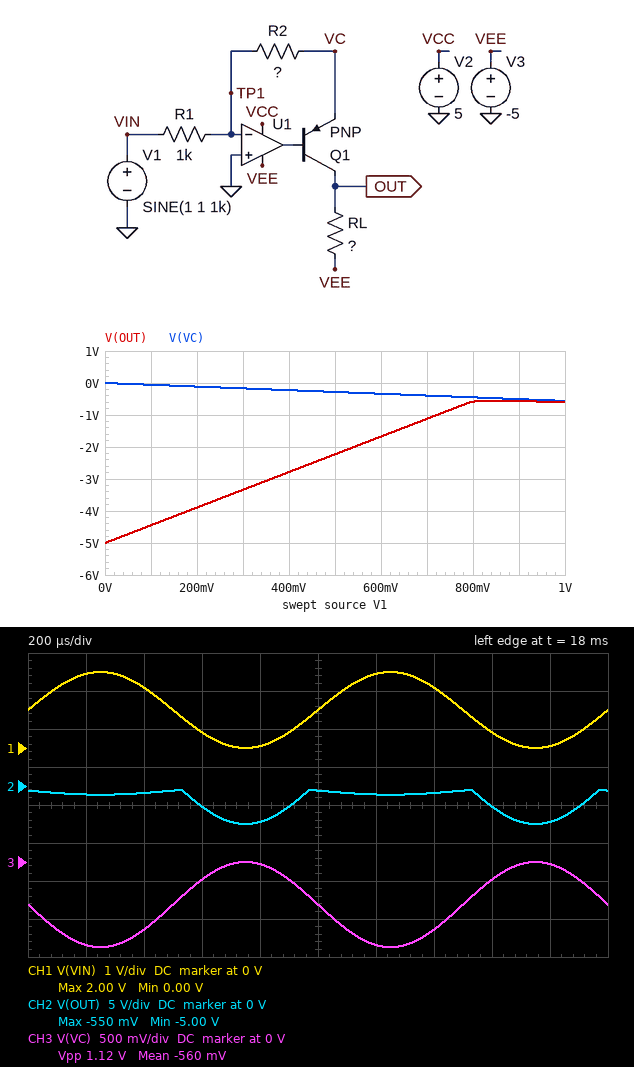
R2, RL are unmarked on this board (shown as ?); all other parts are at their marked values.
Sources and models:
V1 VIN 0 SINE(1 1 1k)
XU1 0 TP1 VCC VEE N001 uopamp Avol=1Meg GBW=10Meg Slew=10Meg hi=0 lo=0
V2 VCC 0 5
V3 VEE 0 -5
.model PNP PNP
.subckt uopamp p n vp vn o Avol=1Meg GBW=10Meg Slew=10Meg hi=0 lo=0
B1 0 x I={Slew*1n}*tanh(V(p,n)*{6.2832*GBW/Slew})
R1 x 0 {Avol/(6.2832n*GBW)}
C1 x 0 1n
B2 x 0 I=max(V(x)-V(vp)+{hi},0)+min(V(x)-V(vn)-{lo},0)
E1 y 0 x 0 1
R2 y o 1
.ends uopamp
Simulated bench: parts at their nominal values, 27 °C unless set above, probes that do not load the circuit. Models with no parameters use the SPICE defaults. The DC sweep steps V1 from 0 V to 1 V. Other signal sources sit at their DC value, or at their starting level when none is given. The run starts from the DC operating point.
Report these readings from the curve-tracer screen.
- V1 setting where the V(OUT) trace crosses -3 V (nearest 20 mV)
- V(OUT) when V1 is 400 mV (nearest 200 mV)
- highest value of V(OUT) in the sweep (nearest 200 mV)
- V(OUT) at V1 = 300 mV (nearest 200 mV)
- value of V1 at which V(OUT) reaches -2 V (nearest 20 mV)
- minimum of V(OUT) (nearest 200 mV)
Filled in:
360 mV
-2.8 V
-600 mV
-3.4 V
540 mV
-5.0 V
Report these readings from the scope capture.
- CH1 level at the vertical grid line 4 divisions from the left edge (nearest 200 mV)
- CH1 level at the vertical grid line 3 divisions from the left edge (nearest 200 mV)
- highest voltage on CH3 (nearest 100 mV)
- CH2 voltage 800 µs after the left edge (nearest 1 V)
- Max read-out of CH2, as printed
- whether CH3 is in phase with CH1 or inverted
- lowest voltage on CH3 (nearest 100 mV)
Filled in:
0 V
400 mV
0 V
-5 V
-550 mV
inverted
-1.1 V
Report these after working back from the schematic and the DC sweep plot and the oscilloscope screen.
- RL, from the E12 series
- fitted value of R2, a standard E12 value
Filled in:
5.6 kΩ
560 Ω
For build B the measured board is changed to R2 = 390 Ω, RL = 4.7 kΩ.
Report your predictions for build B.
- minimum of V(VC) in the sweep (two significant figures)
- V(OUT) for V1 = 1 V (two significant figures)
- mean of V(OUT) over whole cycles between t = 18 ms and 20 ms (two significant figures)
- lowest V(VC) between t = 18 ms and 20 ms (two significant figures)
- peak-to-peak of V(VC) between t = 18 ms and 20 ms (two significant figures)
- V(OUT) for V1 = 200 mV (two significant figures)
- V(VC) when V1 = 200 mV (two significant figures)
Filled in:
-390 mV
-480 mV
-2.0 V
-780 mV
780 mV
-4.1 V
-78 mV
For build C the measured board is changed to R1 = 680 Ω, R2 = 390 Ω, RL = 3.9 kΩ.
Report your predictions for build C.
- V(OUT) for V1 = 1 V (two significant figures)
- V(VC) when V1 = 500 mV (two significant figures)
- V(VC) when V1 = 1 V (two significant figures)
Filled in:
-620 mV
-290 mV
-570 mV
